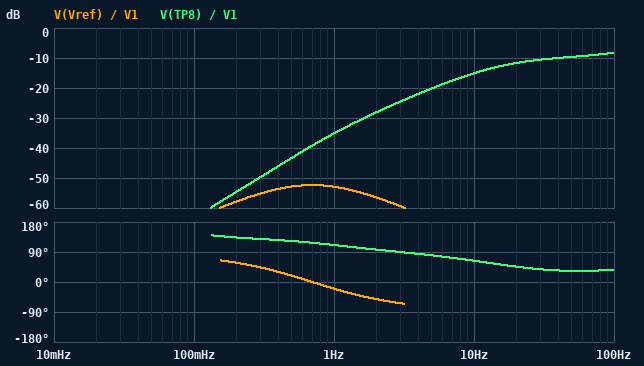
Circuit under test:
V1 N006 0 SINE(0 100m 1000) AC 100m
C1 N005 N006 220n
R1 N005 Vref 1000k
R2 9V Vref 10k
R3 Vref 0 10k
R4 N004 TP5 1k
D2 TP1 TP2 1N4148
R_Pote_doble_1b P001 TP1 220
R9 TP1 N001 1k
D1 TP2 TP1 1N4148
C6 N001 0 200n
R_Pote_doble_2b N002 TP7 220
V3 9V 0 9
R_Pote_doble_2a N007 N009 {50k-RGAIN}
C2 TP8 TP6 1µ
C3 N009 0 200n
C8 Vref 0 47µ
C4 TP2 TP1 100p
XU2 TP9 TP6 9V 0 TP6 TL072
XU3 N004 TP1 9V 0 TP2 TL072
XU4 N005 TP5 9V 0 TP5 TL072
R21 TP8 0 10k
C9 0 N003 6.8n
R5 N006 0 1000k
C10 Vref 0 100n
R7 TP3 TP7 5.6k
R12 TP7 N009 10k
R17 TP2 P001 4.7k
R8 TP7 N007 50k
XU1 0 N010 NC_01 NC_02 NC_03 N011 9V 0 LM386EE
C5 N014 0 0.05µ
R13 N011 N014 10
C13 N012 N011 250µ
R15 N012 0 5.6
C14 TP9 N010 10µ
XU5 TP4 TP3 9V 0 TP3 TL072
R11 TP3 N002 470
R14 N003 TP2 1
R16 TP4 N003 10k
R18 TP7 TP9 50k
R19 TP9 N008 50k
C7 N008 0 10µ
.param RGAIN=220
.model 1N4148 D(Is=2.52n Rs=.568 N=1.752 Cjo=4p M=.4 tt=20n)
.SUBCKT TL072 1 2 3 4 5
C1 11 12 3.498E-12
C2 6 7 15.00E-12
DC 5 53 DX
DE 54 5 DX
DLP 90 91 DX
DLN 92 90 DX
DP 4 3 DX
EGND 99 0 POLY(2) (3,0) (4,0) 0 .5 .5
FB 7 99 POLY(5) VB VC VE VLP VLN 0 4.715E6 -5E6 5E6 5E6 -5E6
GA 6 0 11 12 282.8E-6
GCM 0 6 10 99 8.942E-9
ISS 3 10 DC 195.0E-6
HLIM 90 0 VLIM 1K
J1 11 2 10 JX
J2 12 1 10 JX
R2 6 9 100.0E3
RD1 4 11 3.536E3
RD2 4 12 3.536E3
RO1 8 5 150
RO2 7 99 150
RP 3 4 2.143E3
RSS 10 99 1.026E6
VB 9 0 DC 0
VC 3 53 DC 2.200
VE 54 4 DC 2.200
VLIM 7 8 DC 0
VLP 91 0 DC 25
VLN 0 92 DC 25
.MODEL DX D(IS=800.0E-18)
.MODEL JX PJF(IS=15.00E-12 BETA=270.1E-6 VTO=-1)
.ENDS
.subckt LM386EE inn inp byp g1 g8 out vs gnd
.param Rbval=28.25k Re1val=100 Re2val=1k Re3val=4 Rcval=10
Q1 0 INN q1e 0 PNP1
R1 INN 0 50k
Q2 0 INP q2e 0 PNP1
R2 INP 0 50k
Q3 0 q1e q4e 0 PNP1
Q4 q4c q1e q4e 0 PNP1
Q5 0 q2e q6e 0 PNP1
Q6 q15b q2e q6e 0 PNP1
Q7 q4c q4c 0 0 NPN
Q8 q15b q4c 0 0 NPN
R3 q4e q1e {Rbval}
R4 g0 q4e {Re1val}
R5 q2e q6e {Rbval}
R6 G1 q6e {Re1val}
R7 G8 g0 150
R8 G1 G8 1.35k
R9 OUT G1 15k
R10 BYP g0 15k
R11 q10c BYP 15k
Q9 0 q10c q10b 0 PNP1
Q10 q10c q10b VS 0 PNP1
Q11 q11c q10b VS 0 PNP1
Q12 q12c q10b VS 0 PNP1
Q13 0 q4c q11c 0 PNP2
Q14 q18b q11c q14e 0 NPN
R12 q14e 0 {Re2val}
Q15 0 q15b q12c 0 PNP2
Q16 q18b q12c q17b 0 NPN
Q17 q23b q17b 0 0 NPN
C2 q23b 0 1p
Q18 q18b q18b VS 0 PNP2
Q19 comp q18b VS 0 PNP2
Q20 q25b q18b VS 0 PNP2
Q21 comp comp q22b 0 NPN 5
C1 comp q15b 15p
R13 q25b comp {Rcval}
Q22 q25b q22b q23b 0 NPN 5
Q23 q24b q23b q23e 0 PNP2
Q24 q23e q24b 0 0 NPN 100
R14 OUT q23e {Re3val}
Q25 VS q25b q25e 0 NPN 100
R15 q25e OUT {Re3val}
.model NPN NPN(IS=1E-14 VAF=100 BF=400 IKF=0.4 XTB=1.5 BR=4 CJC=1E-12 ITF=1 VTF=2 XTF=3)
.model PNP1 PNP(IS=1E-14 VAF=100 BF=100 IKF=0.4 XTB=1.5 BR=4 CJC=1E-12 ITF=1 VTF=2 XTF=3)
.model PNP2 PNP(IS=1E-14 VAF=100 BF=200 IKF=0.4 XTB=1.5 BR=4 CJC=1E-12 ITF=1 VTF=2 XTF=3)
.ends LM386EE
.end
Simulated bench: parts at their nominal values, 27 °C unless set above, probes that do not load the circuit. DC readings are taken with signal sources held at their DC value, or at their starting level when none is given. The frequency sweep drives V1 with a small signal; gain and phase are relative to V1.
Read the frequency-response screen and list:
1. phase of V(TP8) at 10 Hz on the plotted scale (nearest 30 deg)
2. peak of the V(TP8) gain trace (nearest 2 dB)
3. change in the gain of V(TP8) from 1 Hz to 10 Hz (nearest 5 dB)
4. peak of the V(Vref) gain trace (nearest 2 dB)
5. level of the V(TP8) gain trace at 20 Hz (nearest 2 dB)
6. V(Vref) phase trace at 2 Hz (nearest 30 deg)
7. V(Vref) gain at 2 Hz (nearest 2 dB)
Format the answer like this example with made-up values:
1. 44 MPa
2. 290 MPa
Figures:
1. 60 deg
2. -8 dB
3. 20 dB
4. -52 dB
5. -12 dB
6. -60 deg
7. -56 dB
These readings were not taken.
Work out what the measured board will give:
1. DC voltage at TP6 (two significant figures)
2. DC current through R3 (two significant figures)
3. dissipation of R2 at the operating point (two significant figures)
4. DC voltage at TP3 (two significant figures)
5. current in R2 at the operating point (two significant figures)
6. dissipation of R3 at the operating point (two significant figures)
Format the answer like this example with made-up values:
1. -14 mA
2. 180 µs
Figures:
1. 4.5 V
2. 450 µA
3. 2.0 mW
4. 4.5 V
5. 450 µA
6. 2.0 mW
